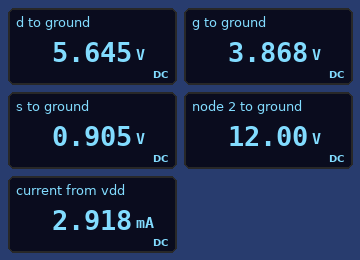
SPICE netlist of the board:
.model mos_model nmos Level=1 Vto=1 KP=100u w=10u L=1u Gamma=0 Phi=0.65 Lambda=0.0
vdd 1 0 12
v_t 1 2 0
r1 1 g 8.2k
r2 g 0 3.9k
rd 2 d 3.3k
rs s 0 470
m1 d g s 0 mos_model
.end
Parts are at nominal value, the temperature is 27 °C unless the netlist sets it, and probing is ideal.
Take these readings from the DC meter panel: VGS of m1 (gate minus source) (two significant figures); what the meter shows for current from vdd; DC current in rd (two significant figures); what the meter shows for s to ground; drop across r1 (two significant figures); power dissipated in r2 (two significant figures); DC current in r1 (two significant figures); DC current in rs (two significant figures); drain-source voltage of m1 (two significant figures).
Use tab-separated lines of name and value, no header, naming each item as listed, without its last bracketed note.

VGS of m1 (gate minus source)	3.0 V
what the meter shows for current from vdd	2.918 mA
DC current in rd	1.9 mA
what the meter shows for s to ground	0.905 V
drop across r1	8.1 V
power dissipated in r2	3.8 mW
DC current in r1	990 µA
DC current in rs	1.9 mA
drain-source voltage of m1	4.7 V
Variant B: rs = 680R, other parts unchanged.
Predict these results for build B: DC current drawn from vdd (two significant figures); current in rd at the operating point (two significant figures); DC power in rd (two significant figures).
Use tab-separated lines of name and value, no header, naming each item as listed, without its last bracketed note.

DC current drawn from vdd	2.6 mA
current in rd at the operating point	1.6 mA
DC power in rd	8.4 mW
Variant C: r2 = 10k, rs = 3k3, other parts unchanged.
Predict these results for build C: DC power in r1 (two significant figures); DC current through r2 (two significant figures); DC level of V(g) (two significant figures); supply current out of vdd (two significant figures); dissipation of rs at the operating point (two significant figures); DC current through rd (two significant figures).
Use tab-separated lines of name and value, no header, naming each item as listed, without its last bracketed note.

DC power in r1	3.6 mW
DC current through r2	660 µA
DC level of V(g)	6.6 V
supply current out of vdd	1.9 mA
dissipation of rs at the operating point	4.9 mW
DC current through rd	1.2 mA
